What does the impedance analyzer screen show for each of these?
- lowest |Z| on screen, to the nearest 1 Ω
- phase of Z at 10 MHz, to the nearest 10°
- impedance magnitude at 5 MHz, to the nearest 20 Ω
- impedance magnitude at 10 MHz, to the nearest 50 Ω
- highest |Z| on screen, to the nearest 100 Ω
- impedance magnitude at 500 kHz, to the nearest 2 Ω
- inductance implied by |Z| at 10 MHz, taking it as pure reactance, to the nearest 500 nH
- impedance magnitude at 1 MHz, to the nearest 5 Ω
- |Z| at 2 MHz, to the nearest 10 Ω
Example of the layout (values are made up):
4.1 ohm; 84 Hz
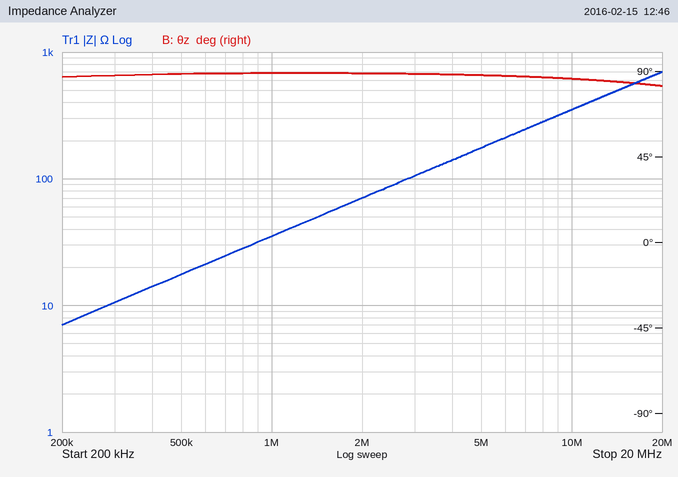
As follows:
7 Ω; 90°; 180 Ω; 350 Ω; 700 Ω; 18 Ω; 5.5 µH; 35 Ω; 70 Ω
